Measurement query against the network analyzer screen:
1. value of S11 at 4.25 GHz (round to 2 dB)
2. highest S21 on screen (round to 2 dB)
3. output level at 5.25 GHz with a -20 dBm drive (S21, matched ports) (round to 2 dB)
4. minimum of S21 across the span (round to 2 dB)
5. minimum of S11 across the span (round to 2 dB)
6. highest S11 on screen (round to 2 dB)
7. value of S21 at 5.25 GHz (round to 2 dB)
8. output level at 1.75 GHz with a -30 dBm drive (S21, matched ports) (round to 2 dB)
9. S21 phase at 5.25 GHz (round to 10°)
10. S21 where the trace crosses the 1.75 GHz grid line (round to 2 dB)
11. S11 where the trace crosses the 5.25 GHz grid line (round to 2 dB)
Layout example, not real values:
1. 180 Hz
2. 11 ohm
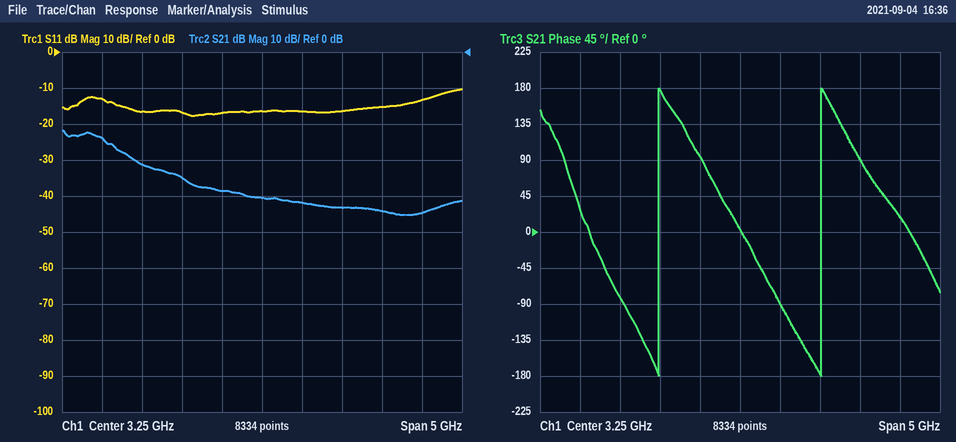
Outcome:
1. -16 dB
2. -22 dB
3. -64 dBm
4. -46 dB
5. -18 dB
6. -10 dB
7. -44 dB
8. -62 dBm
9. 20°
10. -32 dB
11. -14 dB
